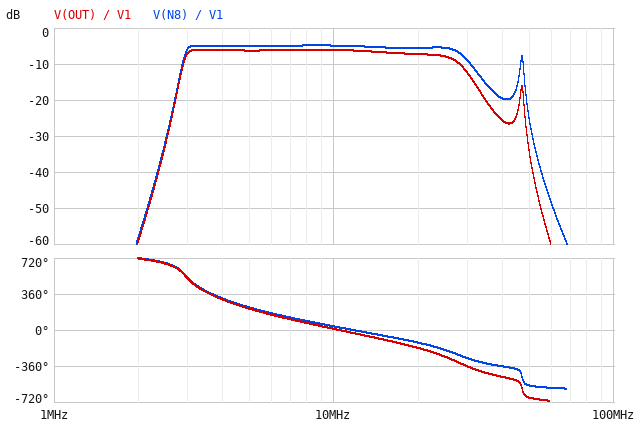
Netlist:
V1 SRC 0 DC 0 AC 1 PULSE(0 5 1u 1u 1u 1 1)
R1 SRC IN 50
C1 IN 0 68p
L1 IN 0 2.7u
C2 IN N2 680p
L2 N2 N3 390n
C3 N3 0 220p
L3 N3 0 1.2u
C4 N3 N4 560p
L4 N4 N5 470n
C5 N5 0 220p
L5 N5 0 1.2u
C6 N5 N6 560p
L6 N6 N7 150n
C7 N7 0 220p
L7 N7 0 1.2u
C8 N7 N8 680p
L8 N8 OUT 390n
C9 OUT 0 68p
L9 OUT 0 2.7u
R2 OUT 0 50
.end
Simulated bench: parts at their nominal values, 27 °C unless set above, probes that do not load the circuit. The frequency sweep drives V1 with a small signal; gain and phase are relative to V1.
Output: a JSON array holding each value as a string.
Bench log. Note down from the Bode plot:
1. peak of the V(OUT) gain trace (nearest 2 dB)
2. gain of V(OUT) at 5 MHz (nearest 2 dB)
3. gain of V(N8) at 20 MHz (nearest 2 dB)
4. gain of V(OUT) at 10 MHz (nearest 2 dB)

["-6 dB", "-6 dB", "-6 dB", "-6 dB"]
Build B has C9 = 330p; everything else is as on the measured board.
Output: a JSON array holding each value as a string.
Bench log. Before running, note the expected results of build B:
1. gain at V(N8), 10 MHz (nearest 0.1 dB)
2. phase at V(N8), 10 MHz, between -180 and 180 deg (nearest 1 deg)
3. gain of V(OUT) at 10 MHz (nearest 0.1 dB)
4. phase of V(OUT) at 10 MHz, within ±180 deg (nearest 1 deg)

["-9.0 dB", "27 deg", "-7.1 dB", "-11 deg"]
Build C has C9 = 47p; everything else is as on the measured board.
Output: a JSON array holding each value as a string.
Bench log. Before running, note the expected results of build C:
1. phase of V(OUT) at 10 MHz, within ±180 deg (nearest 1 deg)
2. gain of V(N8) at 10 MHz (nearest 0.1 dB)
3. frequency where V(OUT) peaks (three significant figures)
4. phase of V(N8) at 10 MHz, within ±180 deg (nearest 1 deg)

["13 deg", "-4.6 dB", "8.54 MHz", "38 deg"]
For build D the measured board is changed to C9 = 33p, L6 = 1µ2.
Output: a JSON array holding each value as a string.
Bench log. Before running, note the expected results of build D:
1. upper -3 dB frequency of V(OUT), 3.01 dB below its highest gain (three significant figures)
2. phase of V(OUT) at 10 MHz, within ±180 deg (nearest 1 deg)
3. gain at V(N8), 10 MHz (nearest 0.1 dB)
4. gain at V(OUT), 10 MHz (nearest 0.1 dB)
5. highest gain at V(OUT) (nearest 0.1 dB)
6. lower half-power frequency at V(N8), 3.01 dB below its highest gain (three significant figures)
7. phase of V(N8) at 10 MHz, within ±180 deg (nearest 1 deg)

["20.0 MHz", "-20 deg", "-5.8 dB", "-7.4 dB", "-6.2 dB", "2.80 MHz", "4 deg"]
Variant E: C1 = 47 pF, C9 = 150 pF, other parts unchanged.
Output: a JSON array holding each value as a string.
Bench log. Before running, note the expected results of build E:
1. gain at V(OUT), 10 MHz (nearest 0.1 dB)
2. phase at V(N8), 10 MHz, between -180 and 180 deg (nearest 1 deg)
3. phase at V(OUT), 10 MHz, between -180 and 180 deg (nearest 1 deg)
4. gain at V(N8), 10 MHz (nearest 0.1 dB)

["-6.2 dB", "34 deg", "6 deg", "-5.9 dB"]
